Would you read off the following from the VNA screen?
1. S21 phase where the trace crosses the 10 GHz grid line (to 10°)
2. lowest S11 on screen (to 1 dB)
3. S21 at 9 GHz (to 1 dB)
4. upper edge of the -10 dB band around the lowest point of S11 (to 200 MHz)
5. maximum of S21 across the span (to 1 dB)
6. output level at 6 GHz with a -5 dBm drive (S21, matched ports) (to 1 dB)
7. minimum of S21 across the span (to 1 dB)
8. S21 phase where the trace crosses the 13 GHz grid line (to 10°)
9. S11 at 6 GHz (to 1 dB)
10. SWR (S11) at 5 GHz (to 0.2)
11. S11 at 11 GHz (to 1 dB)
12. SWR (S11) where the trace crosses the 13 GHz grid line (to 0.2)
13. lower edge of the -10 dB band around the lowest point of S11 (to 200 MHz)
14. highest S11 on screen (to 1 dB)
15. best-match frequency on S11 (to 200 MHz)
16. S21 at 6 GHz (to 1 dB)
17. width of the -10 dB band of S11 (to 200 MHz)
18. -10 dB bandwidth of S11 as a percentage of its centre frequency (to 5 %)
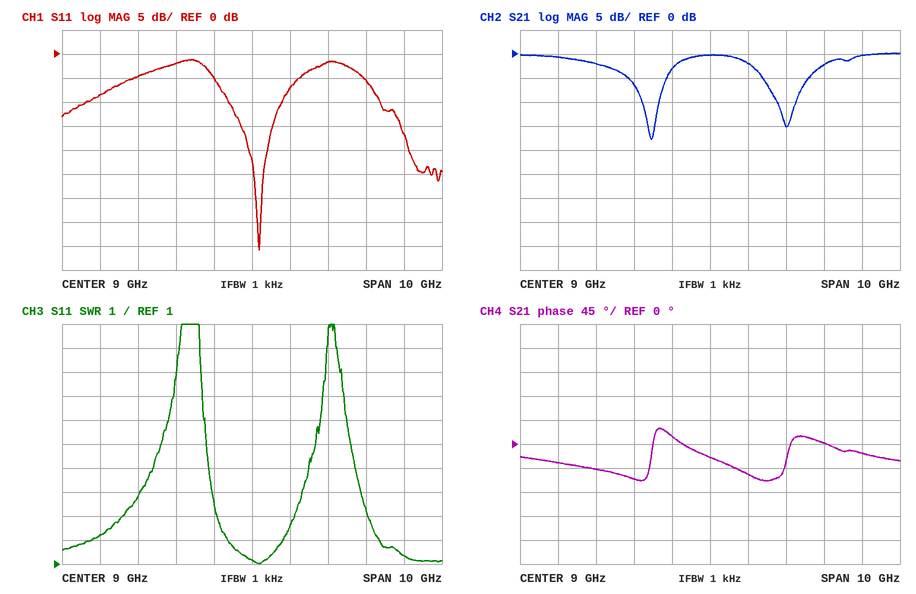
-60°
-41 dB
0 dB
9.8 GHz
0 dB
-7 dBm
-18 dB
-20°
-5 dB
2.2
-2 dB
1.4
8.4 GHz
-1 dB
9.2 GHz
-2 dB
1.4 GHz
15 %
